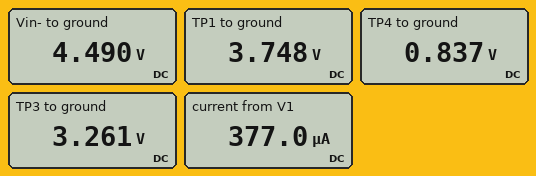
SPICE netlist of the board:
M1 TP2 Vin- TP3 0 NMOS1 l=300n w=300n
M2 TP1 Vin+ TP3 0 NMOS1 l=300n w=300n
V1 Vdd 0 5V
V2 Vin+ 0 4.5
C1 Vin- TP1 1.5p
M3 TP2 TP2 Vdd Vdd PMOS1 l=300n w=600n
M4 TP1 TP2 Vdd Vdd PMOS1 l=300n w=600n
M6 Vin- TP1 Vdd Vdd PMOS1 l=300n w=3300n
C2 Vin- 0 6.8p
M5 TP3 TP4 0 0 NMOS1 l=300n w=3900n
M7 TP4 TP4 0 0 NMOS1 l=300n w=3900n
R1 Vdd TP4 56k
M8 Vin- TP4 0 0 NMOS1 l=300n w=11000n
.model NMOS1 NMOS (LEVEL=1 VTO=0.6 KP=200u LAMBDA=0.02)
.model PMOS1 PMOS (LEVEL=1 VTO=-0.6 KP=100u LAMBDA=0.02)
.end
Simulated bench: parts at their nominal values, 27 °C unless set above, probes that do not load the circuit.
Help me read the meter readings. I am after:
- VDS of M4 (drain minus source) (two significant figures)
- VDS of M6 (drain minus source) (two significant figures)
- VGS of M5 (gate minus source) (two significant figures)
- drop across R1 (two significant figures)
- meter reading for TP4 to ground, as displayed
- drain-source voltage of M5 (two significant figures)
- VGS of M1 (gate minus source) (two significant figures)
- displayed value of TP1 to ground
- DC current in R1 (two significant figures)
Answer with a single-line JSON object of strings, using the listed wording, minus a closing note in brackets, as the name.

{"VDS of M4 (drain minus source)": "-1.3 V", "VDS of M6 (drain minus source)": "-510 mV", "VGS of M5 (gate minus source)": "840 mV", "drop across R1": "4.2 V", "meter reading for TP4 to ground, as displayed": "0.837 V", "drain-source voltage of M5": "3.3 V", "VGS of M1 (gate minus source)": "1.2 V", "displayed value of TP1 to ground": "3.748 V", "DC current in R1": "74 µA"}
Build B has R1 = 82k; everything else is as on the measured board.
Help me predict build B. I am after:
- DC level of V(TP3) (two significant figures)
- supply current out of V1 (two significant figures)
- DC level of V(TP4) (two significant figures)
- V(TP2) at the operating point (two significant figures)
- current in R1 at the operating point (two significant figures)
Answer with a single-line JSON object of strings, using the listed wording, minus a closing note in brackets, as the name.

{"DC level of V(TP3)": "3.4 V", "supply current out of V1": "260 µA", "DC level of V(TP4)": "800 mV", "V(TP2) at the operating point": "3.9 V", "current in R1 at the operating point": "51 µA"}
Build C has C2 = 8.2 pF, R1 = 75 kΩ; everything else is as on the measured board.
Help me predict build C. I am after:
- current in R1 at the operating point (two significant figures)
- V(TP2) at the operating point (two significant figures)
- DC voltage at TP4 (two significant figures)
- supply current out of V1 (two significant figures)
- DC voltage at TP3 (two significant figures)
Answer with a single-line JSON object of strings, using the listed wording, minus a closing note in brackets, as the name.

{"current in R1 at the operating point": "56 µA", "V(TP2) at the operating point": "3.9 V", "DC voltage at TP4": "810 mV", "supply current out of V1": "280 µA", "DC voltage at TP3": "3.4 V"}
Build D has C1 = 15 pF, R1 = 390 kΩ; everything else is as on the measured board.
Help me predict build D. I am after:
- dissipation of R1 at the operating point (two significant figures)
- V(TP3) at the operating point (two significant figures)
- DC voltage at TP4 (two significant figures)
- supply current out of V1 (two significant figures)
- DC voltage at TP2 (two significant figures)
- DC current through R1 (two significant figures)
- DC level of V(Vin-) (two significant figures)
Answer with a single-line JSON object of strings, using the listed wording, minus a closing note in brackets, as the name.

{"dissipation of R1 at the operating point": "48 µW", "V(TP3) at the operating point": "3.7 V", "DC voltage at TP4": "690 mV", "supply current out of V1": "56 µA", "DC voltage at TP2": "4.2 V", "DC current through R1": "11 µA", "DC level of V(Vin-)": "4.5 V"}
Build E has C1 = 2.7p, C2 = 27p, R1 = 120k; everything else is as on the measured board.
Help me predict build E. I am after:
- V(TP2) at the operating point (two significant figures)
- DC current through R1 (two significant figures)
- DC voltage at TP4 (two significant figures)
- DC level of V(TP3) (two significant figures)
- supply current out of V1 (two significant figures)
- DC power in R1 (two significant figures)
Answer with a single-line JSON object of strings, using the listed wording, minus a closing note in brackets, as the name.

{"V(TP2) at the operating point": "4.0 V", "DC current through R1": "35 µA", "DC voltage at TP4": "760 mV", "DC level of V(TP3)": "3.5 V", "supply current out of V1": "180 µA", "DC power in R1": "150 µW"}
